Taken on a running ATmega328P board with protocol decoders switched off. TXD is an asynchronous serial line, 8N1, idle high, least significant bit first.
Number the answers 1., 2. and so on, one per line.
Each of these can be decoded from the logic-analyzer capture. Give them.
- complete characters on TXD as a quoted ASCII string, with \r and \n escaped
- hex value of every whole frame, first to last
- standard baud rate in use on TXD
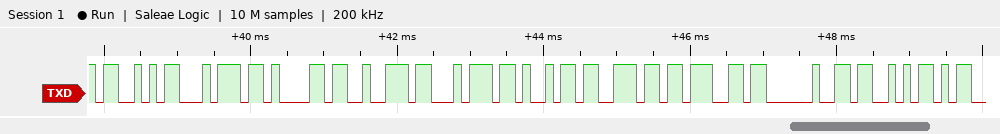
1. "Starting S"
2. 0x53 0x74 0x61 0x72 0x74 0x69 0x6E 0x67 0x20 0x53
3. 9600 baud
